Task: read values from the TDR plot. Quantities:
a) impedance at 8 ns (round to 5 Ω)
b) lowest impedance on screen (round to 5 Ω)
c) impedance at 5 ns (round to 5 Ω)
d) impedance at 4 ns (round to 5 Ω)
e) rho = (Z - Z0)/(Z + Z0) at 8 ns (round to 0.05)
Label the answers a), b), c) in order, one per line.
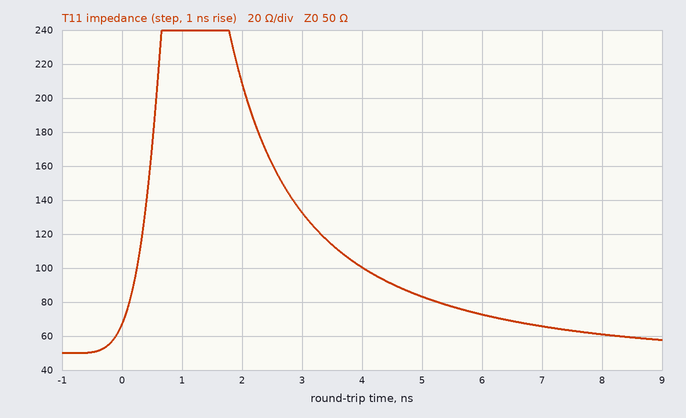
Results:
a) 60 Ω
b) 50 Ω
c) 85 Ω
d) 100 Ω
e) +0.10
